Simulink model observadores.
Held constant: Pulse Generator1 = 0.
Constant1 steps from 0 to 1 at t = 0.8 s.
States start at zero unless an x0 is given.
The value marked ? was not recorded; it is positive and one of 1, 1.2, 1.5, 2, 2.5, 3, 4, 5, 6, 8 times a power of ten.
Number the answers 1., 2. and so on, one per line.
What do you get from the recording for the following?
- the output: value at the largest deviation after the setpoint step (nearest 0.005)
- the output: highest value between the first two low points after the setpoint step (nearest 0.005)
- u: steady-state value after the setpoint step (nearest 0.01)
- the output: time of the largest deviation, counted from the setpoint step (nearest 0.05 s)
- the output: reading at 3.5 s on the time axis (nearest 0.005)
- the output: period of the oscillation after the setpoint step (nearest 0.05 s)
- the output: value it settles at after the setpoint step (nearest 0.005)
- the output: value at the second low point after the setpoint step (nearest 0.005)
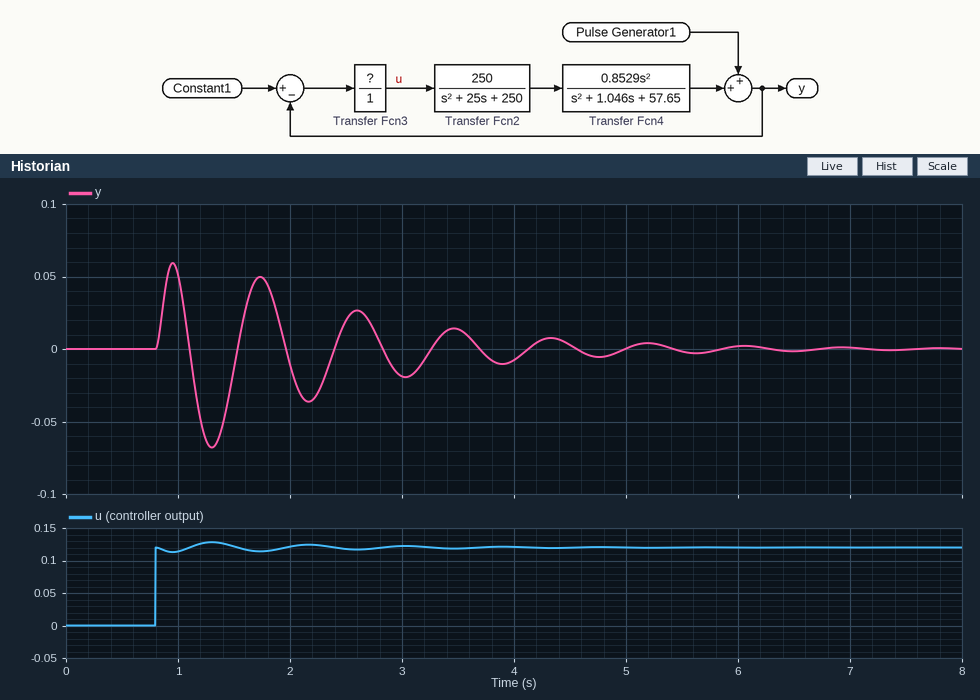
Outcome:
1. -0.070
2. 0.050
3. 0.12
4. 0.50 s
5. 0.015
6. 0.85 s
7. 0.000
8. -0.035
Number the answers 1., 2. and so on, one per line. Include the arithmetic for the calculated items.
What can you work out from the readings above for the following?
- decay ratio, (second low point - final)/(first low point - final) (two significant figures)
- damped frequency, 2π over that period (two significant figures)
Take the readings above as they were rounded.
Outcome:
1. (-0.035 - 0) / (-0.07 - 0) = 0.50
2. 2π / 0.85 = 7.4 rad/s
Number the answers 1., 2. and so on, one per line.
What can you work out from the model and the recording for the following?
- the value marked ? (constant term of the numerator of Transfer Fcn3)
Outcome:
1. 0.12
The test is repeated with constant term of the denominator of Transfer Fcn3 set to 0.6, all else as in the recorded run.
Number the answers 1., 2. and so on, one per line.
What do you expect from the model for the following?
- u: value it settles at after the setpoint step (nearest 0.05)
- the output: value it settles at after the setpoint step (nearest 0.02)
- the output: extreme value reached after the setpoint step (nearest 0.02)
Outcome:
1. 0.20
2. 0.00
3. -0.10
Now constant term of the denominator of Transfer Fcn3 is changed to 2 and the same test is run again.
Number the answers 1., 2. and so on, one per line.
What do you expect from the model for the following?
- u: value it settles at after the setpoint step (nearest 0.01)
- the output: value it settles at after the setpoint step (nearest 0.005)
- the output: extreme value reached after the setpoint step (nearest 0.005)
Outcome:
1. 0.06
2. 0.000
3. -0.035
